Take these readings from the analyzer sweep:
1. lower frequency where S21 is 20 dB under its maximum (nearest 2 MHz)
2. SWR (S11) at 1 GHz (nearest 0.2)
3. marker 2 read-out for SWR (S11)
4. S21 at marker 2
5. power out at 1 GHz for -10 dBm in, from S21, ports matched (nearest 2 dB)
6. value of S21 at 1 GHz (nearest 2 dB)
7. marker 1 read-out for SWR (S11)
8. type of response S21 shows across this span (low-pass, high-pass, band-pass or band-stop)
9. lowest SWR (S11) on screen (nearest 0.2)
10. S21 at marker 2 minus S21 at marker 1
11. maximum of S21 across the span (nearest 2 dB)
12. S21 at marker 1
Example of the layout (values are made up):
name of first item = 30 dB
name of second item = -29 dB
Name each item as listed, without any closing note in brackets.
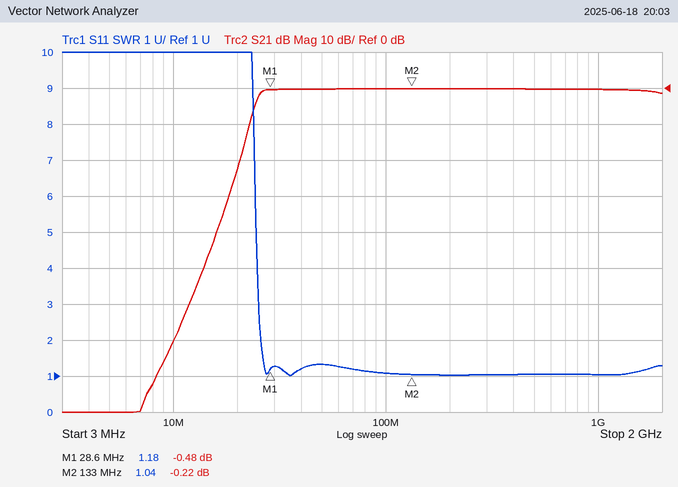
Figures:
lower frequency where S21 is 20 dB under its maximum = 20 MHz
SWR (S11) at 1 GHz = 1.0
marker 2 read-out for SWR = 1.04
S21 at marker 2 = -0.22 dB
power out at 1 GHz for -10 dBm in, from S21, ports matched = -10 dBm
value of S21 at 1 GHz = 0 dB
marker 1 read-out for SWR = 1.18
type of response S21 shows across this span = high-pass
lowest SWR (S11) on screen = 1.0
S21 at marker 2 minus S21 at marker 1 = 0.26 dB
maximum of S21 across the span = 0 dB
S21 at marker 1 = -0.48 dB
